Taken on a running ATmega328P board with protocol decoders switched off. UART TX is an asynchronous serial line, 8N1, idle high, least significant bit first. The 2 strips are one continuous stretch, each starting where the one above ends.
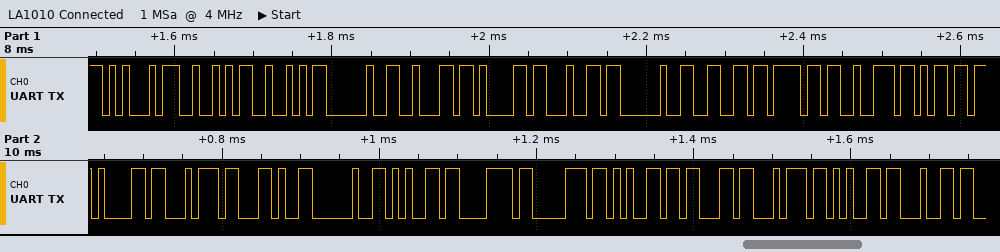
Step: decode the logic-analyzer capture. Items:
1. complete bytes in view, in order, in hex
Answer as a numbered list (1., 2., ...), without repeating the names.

1. 0x45 0x52 0x52 0x20 0x62 0x61 0x64 0x20 0x66 0x6F 0x72 0x6D 0x61 0x74 0x2C 0x20 0x65 0x78 0x70 0x65 0x63 0x74 0x65 0x64
